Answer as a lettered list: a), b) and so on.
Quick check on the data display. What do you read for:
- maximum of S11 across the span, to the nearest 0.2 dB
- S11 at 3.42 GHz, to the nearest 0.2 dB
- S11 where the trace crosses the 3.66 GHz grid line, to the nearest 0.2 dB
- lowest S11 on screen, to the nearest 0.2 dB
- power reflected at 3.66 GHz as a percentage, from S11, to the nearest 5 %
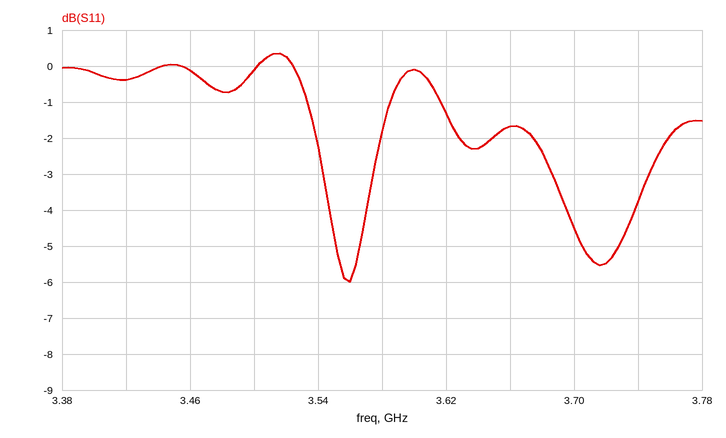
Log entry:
a) 0.4 dB
b) -0.4 dB
c) -1.6 dB
d) -6.0 dB
e) 70 %
